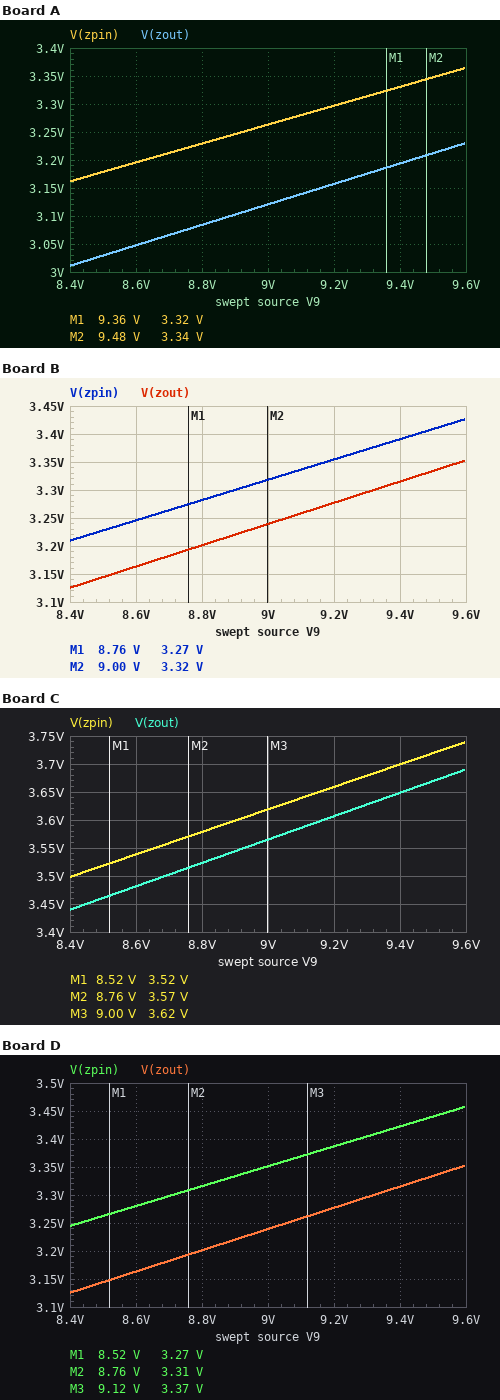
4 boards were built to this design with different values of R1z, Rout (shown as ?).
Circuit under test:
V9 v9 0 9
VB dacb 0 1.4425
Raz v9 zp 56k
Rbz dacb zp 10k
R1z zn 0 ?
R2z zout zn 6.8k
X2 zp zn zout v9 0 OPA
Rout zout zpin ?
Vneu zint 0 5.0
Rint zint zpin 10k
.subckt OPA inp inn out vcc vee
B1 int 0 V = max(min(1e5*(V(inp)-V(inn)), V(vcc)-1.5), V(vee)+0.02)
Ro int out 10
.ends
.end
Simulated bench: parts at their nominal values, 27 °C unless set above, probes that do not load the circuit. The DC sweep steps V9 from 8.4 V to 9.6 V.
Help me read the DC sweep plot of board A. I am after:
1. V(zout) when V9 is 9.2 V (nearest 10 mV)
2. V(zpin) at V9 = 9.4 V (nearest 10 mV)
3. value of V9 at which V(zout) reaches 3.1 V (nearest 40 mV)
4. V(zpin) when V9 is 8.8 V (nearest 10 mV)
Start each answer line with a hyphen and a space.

- 3.16 V
- 3.33 V
- 8.88 V
- 3.23 V
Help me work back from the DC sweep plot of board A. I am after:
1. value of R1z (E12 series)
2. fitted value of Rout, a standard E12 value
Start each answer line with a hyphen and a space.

- 33 kΩ
- 820 Ω
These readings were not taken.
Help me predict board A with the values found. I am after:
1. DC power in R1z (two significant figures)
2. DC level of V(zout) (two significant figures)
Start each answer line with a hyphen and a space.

- 200 µW
- 3.1 V
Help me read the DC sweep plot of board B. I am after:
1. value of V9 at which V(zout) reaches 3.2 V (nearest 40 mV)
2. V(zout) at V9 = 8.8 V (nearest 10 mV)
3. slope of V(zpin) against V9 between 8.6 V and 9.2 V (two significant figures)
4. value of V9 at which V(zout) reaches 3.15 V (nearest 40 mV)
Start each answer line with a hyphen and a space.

- 8.80 V
- 3.20 V
- 0.18 V/V
- 8.52 V
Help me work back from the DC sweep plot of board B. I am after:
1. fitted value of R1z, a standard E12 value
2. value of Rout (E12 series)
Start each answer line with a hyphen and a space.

- 27 kΩ
- 470 Ω
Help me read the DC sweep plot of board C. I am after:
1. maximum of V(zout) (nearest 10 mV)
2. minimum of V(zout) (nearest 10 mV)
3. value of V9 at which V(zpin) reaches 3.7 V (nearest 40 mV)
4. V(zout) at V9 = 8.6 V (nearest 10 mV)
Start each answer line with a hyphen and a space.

- 3.69 V
- 3.44 V
- 9.40 V
- 3.48 V
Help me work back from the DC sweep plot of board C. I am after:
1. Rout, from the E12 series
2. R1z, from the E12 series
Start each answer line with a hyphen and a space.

- 390 Ω
- 18 kΩ
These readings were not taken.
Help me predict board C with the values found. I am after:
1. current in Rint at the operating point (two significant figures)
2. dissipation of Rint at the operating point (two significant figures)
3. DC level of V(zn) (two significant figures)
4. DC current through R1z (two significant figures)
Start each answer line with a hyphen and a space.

- 140 µA
- 190 µW
- 2.6 V
- 140 µA
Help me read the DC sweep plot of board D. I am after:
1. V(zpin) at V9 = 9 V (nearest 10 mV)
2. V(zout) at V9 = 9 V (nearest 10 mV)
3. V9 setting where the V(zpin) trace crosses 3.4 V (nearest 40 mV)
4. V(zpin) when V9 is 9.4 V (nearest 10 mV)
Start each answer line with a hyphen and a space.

- 3.35 V
- 3.24 V
- 9.28 V
- 3.42 V
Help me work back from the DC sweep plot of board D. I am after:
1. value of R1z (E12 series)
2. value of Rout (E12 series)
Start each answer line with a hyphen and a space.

- 27 kΩ
- 680 Ω
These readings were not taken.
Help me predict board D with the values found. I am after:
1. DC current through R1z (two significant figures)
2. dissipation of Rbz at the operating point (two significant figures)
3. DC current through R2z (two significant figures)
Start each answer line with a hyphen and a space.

- 96 µA
- 130 µW
- 96 µA
